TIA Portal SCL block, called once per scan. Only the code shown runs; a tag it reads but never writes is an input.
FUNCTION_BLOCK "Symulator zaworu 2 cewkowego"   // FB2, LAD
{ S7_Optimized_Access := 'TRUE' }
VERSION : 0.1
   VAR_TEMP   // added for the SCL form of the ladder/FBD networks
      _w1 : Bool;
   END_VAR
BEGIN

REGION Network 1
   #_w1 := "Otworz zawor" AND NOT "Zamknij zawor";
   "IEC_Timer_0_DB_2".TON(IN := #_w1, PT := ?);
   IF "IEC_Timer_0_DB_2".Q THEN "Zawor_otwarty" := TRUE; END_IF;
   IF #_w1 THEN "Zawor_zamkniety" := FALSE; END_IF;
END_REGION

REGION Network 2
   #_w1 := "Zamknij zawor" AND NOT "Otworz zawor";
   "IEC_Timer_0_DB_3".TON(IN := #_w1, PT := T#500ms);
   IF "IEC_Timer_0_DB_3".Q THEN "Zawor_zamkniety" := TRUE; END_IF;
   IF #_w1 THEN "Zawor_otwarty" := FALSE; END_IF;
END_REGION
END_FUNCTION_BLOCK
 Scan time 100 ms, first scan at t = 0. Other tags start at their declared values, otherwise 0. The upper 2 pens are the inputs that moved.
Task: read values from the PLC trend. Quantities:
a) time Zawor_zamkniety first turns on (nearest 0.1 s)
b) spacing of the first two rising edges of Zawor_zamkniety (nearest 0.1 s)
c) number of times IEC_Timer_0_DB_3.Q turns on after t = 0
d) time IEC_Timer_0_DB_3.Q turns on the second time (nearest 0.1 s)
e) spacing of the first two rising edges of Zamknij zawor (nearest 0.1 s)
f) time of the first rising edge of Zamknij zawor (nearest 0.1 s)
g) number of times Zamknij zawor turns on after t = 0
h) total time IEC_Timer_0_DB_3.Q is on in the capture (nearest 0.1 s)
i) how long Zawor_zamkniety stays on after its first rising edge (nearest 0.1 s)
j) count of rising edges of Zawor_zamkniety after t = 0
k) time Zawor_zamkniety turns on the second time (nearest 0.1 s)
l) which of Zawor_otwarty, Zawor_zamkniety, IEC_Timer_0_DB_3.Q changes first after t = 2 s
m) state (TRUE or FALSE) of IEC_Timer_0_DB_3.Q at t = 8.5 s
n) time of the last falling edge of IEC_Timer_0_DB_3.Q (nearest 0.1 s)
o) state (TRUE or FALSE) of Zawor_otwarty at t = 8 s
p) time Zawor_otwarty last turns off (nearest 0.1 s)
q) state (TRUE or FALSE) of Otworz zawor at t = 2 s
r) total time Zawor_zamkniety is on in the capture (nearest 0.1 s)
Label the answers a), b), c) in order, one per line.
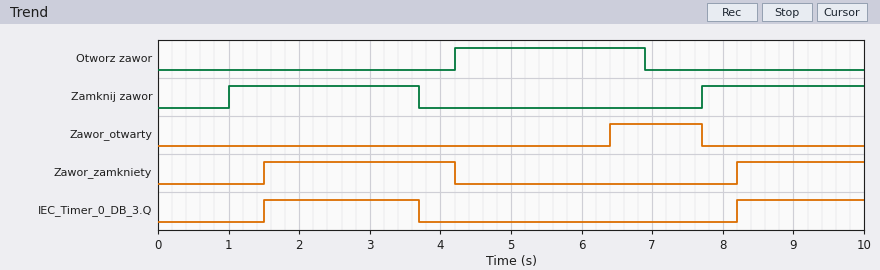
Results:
a) 1.5 s
b) 6.7 s
c) 2
d) 8.2 s
e) 6.7 s
f) 1.0 s
g) 2
h) 4.0 s
i) 2.7 s
j) 2
k) 8.2 s
l) IEC_Timer_0_DB_3.Q
m) TRUE
n) 3.7 s
o) FALSE
p) 7.7 s
q) FALSE
r) 4.5 s
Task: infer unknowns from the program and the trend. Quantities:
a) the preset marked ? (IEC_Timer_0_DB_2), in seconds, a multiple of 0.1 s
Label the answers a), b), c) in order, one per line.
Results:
a) 2.2 s
